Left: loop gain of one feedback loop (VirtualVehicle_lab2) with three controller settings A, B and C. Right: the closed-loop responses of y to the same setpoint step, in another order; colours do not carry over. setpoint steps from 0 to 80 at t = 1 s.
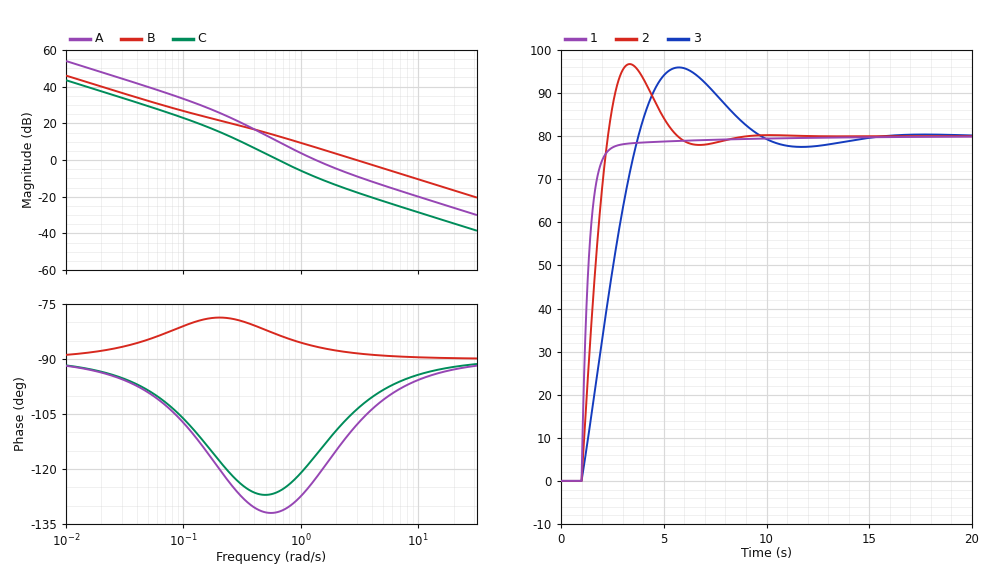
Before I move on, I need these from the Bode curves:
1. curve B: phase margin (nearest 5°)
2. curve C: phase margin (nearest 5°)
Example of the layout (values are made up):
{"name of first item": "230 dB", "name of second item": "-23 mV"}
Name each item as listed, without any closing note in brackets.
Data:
{"curve B: phase margin": "90°", "curve C: phase margin": "55°"}
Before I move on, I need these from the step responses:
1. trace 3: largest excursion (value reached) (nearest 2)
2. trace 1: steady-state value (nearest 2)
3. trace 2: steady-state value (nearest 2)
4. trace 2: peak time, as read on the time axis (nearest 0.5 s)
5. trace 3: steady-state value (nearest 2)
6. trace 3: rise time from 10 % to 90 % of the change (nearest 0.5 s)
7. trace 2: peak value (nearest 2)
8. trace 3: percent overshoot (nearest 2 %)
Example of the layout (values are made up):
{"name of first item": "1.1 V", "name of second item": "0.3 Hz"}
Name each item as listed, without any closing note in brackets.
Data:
{"trace 3: largest excursion (value reached)": "96", "trace 1: steady-state value": "80", "trace 2: steady-state value": "80", "trace 2: peak time, as read on the time axis": "3.5 s", "trace 3: steady-state value": "80", "trace 3: rise time from 10 % to 90 % of the change": "2.0 s", "trace 2: peak value": "96", "trace 3: percent overshoot": "20 %"}
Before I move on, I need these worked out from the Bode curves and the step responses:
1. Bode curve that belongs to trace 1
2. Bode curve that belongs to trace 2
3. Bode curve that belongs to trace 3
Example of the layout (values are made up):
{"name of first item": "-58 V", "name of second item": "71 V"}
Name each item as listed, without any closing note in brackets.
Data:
{"Bode curve that belongs to trace 1": "B", "Bode curve that belongs to trace 2": "A", "Bode curve that belongs to trace 3": "C"}
